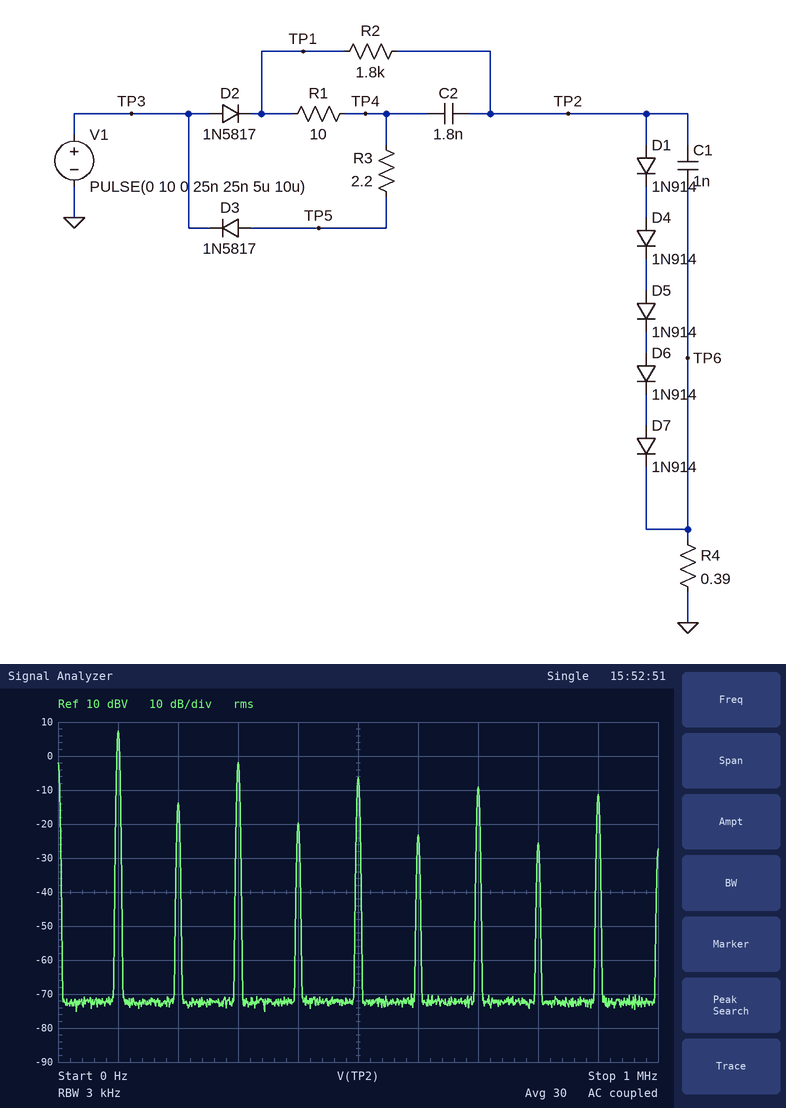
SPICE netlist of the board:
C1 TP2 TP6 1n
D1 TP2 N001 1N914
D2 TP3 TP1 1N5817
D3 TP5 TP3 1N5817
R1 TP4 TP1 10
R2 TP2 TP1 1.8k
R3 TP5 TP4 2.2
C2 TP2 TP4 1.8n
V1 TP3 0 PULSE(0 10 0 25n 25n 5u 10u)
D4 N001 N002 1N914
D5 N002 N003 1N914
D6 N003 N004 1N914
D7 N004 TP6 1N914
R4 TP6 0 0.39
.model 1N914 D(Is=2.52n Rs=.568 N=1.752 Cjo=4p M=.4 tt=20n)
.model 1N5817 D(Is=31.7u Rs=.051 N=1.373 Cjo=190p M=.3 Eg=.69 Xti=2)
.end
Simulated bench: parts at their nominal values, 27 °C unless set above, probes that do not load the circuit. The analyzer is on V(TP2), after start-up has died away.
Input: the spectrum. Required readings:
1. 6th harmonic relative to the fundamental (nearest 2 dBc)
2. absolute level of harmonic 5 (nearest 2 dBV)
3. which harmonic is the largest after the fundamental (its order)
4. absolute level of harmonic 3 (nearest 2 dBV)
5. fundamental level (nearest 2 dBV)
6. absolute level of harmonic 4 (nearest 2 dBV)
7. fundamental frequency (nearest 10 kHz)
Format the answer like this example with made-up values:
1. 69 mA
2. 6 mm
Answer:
1. -30 dBc
2. -6 dBV
3. 3
4. -2 dBV
5. 8 dBV
6. -20 dBV
7. 100 kHz
